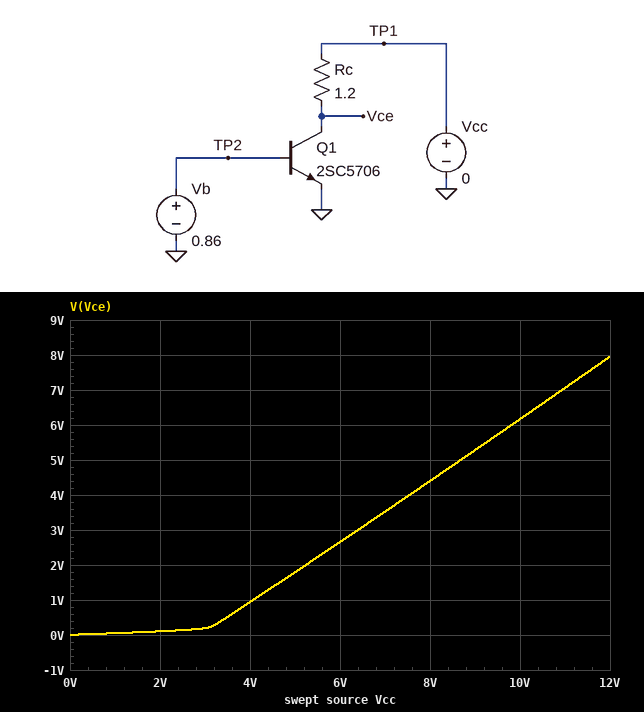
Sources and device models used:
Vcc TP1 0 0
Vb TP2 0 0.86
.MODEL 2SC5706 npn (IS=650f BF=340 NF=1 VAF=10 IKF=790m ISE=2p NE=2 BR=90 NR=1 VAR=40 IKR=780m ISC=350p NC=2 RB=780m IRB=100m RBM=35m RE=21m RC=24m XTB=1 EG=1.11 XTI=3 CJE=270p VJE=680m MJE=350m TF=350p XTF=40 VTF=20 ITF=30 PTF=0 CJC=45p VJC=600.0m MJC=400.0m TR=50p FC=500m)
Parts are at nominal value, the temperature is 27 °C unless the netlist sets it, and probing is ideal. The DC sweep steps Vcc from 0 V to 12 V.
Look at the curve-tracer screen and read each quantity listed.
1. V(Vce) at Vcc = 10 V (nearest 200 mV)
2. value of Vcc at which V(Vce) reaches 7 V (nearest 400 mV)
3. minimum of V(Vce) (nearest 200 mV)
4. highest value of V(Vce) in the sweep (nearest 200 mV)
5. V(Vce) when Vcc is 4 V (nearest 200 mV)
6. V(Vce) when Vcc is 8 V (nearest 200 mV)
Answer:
6.2 V
10.8 V
0 V
8.0 V
1.0 V
4.4 V
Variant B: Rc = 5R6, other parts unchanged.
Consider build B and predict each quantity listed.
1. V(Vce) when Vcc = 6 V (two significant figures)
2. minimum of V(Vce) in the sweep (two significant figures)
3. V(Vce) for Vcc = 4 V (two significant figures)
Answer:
69 mV
5.7 mV
47 mV
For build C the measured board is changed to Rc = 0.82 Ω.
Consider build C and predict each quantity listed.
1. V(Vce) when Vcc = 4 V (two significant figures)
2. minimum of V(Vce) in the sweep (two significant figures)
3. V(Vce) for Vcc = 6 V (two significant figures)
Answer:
1.8 V
5.4 mV
3.6 V
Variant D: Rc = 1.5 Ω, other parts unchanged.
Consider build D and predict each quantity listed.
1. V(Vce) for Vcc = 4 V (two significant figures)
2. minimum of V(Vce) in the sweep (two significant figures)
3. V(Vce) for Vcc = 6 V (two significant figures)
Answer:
320 mV
5.6 mV
2.0 V
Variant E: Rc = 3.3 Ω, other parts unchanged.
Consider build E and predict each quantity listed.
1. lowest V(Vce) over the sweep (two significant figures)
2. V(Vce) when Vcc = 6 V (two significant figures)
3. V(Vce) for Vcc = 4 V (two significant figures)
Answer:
5.7 mV
120 mV
78 mV
